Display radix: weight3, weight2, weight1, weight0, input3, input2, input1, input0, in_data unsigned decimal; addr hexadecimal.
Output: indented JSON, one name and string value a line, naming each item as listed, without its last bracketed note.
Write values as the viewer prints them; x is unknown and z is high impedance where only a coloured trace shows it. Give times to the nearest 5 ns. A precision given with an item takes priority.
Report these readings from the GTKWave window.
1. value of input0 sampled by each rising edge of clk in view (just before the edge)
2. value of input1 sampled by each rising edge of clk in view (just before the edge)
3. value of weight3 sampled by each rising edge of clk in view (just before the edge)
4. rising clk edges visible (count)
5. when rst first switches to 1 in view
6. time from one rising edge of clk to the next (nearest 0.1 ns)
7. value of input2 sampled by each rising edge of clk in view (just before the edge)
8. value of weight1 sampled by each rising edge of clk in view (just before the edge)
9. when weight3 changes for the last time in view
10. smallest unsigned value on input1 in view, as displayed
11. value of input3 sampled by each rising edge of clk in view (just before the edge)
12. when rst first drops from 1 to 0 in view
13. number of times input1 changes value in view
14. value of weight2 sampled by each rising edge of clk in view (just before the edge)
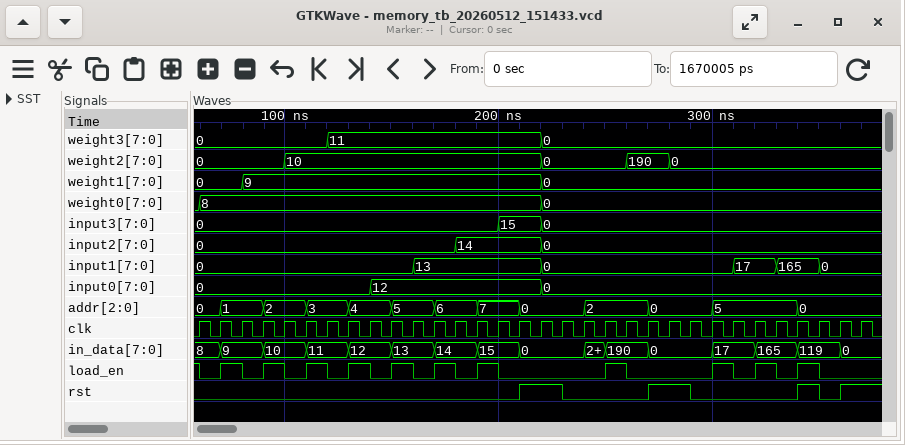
{
  "value of input0 sampled by each rising edge of clk in view": "0, 0, 0, 0, 0, 0, 0, 0, 0, 12, 12, 12, 12, 12, 12, 12, 12, 0, 0, 0, 0, 0, 0, 0, 0, 0, 0, 0, 0, 0, 0, 0",
  "value of input1 sampled by each rising edge of clk in view": "0, 0, 0, 0, 0, 0, 0, 0, 0, 0, 0, 13, 13, 13, 13, 13, 13, 0, 0, 0, 0, 0, 0, 0, 0, 0, 17, 17, 165, 165, 0, 0",
  "value of weight3 sampled by each rising edge of clk in view": "0, 0, 0, 0, 0, 0, 0, 11, 11, 11, 11, 11, 11, 11, 11, 11, 11, 0, 0, 0, 0, 0, 0, 0, 0, 0, 0, 0, 0, 0, 0, 0",
  "rising clk edges visible": "32",
  "when rst first switches to 1 in view": "210 ns",
  "time from one rising edge of clk to the next": "10 ns",
  "value of input2 sampled by each rising edge of clk in view": "0, 0, 0, 0, 0, 0, 0, 0, 0, 0, 0, 0, 0, 14, 14, 14, 14, 0, 0, 0, 0, 0, 0, 0, 0, 0, 0, 0, 0, 0, 0, 0",
  "value of weight1 sampled by each rising edge of clk in view": "0, 0, 0, 9, 9, 9, 9, 9, 9, 9, 9, 9, 9, 9, 9, 9, 9, 0, 0, 0, 0, 0, 0, 0, 0, 0, 0, 0, 0, 0, 0, 0",
  "when weight3 changes for the last time in view": "220 ns",
  "smallest unsigned value on input1 in view, as displayed": "0",
  "value of input3 sampled by each rising edge of clk in view": "0, 0, 0, 0, 0, 0, 0, 0, 0, 0, 0, 0, 0, 0, 0, 15, 15, 0, 0, 0, 0, 0, 0, 0, 0, 0, 0, 0, 0, 0, 0, 0",
  "when rst first drops from 1 to 0 in view": "230 ns",
  "number of times input1 changes value in view": "5",
  "value of weight2 sampled by each rising edge of clk in view": "0, 0, 0, 0, 0, 10, 10, 10, 10, 10, 10, 10, 10, 10, 10, 10, 10, 0, 0, 0, 0, 190, 190, 0, 0, 0, 0, 0, 0, 0, 0, 0"
}
